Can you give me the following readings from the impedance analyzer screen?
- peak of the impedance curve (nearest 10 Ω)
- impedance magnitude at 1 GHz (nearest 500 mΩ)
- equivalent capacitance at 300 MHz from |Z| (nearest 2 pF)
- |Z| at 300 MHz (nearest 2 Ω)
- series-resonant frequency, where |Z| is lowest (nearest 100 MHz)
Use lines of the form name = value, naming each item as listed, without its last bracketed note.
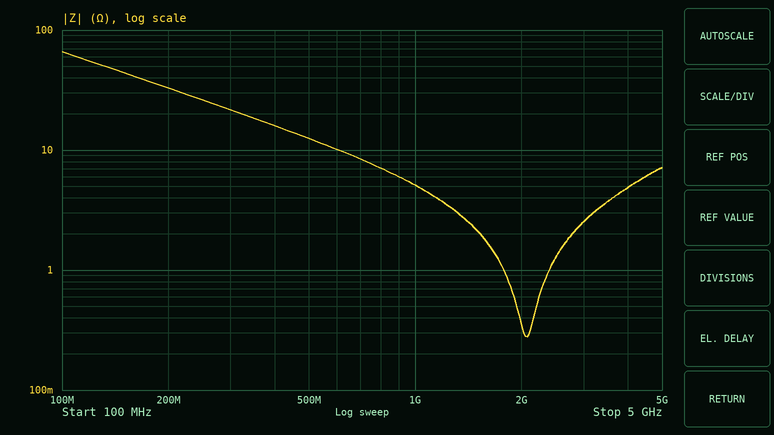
peak of the impedance curve = 70 Ω
impedance magnitude at 1 GHz = 5.0 Ω
equivalent capacitance at 300 MHz from |Z| = 24 pF
|Z| at 300 MHz = 22 Ω
series-resonant frequency, where |Z| is lowest = 2.1 GHz
